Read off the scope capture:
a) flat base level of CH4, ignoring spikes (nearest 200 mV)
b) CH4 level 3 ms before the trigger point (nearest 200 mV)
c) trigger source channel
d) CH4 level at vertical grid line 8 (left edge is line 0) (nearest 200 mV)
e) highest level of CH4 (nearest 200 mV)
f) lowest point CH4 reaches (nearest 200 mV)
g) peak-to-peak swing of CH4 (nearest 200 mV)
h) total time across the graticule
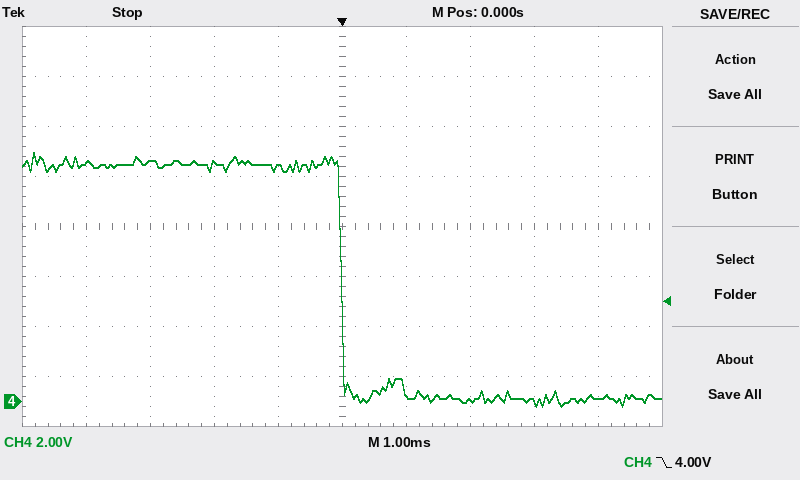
200 mV
9.6 V
CH4
0.0 V
10.0 V
-200 mV
10.2 V
10 ms
